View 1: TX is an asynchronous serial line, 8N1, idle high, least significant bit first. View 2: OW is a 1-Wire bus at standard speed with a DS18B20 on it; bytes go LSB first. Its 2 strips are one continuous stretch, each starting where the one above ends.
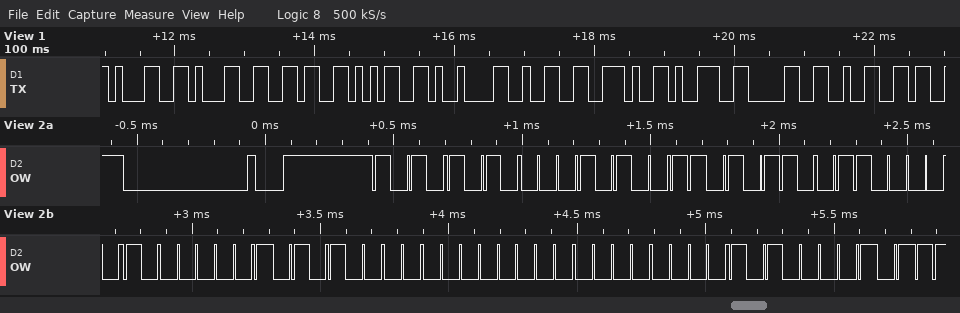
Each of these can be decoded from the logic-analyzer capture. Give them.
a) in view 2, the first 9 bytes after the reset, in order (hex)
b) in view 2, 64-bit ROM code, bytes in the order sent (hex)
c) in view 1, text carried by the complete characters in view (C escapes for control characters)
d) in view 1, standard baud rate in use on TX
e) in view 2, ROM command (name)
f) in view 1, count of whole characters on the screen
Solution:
55 28 6B 06 81 0A 00 00 85
28 6B 06 81 0A 00 00 85
"1165\t2.902"
9600 baud
Match ROM
10
